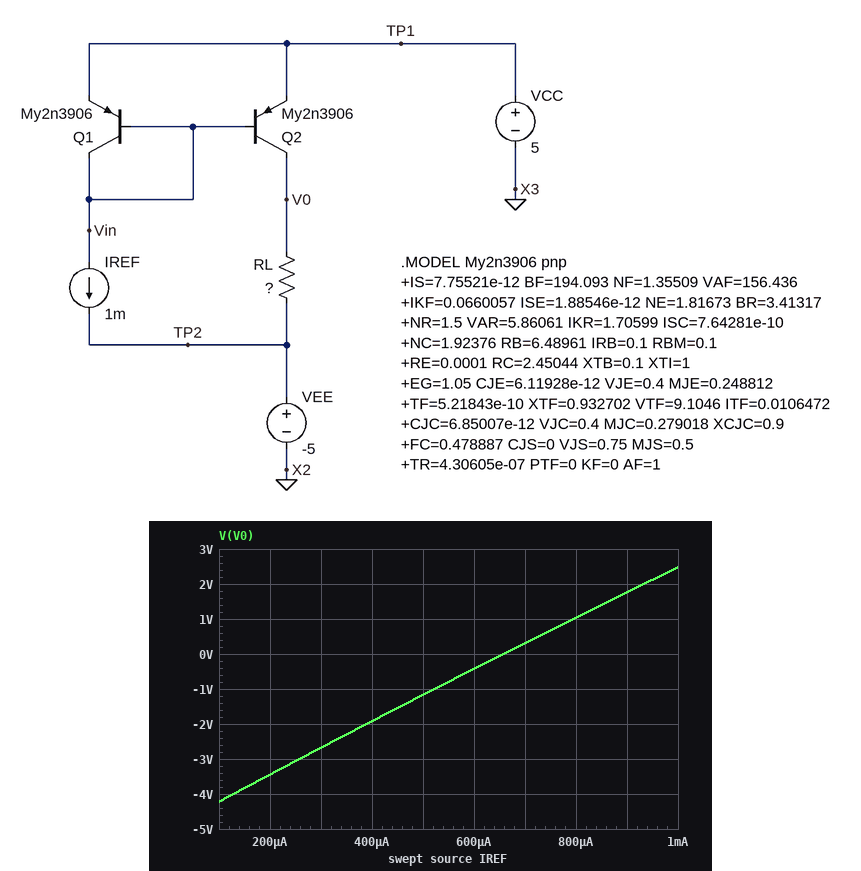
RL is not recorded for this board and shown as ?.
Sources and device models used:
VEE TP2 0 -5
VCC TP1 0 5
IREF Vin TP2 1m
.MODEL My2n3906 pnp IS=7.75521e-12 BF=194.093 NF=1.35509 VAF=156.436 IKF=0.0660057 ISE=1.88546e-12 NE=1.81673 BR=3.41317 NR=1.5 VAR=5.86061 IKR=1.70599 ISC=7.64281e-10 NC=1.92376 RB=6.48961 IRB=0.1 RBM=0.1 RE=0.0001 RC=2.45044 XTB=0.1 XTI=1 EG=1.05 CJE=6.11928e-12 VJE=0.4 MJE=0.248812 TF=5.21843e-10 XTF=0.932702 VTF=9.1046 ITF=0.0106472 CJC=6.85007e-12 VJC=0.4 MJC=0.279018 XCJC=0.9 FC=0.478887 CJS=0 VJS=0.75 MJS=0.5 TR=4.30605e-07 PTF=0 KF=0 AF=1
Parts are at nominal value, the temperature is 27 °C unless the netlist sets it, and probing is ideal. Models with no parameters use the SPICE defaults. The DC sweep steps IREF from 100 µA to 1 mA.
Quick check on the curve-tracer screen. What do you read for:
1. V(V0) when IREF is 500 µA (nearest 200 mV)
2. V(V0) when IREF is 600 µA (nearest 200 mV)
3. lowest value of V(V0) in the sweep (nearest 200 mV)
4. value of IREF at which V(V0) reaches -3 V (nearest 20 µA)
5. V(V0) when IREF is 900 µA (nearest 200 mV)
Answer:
-1.2 V
-400 mV
-4.2 V
260 µA
1.8 V
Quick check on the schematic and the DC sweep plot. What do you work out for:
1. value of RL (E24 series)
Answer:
7.5 kΩ
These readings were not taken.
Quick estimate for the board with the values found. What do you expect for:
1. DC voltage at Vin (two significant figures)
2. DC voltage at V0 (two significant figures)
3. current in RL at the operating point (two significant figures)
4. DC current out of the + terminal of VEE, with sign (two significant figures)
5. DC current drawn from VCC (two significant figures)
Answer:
4.3 V
2.5 V
1.0 mA
-2.0 mA
2.0 mA
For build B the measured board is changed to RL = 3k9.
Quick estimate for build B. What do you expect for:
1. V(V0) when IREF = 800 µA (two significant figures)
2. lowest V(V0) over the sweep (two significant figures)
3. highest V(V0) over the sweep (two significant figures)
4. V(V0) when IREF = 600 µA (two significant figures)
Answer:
-1.8 V
-4.6 V
-1.0 V
-2.6 V
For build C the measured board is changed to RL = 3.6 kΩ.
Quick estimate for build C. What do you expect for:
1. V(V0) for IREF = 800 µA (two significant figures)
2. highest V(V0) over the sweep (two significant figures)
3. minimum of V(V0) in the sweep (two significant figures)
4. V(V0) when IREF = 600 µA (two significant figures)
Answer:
-2.0 V
-1.3 V
-4.6 V
-2.8 V
